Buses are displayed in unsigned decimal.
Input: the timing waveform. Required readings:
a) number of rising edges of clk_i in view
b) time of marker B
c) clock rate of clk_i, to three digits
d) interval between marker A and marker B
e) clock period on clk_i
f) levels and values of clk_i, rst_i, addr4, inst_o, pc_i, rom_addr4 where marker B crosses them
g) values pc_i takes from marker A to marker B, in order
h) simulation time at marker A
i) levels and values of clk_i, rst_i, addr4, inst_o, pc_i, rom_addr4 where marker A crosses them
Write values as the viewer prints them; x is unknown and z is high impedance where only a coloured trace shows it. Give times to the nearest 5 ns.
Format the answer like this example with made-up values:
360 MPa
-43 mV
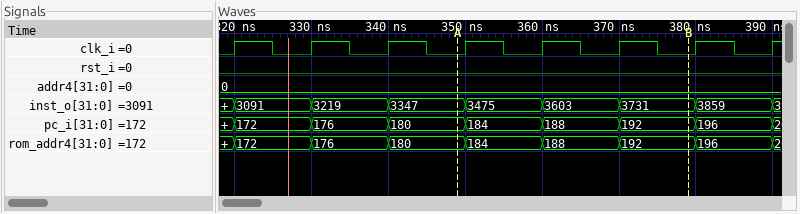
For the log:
8
380 ns
100 MHz
30 ns
10 ns
clk_i=0, rst_i=0, addr4=0, inst_o=3731, pc_i=192, rom_addr4=192
180, 184, 188, 192
350 ns
clk_i=0, rst_i=0, addr4=0, inst_o=3347, pc_i=180, rom_addr4=180
